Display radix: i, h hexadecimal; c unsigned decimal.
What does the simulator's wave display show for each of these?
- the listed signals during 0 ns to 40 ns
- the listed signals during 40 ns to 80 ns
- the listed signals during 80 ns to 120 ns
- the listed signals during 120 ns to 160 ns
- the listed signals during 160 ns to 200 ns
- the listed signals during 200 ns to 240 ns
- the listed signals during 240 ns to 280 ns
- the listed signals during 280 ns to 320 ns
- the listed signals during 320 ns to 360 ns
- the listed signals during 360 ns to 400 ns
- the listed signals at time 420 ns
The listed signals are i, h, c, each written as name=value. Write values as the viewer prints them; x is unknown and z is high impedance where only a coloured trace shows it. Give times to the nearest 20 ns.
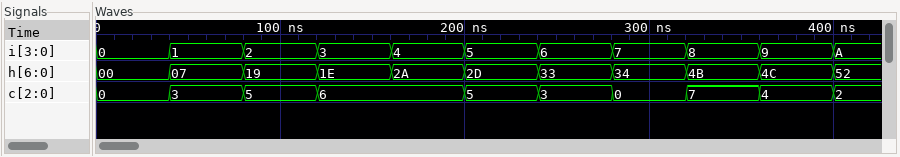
i=0, h=00, c=0
i=1, h=07, c=3
i=2, h=19, c=5
i=3, h=1E, c=6
i=4, h=2A, c=6
i=5, h=2D, c=5
i=6, h=33, c=3
i=7, h=34, c=0
i=8, h=4B, c=7
i=9, h=4C, c=4
i=A, h=52, c=2
